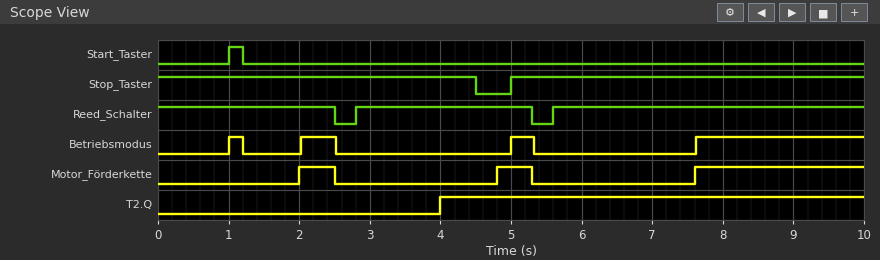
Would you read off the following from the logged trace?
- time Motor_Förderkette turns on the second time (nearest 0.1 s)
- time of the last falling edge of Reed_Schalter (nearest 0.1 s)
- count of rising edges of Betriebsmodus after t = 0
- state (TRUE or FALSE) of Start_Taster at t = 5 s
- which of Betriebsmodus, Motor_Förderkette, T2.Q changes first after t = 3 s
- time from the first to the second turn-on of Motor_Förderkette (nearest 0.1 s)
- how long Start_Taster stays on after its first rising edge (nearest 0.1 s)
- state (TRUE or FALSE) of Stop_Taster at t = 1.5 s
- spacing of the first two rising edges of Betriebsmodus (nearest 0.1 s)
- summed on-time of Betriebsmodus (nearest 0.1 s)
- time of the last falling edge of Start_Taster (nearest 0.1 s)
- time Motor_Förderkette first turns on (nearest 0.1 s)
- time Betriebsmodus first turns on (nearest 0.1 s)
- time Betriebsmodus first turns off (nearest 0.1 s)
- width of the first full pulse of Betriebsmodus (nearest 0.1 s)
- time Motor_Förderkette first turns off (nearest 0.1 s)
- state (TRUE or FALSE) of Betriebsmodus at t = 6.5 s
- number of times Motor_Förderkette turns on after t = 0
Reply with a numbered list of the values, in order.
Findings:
1. 4.8 s
2. 5.3 s
3. 4
4. FALSE
5. T2.Q
6. 2.8 s
7. 0.2 s
8. TRUE
9. 1.0 s
10. 3.4 s
11. 1.2 s
12. 2.0 s
13. 1.0 s
14. 1.2 s
15. 0.2 s
16. 2.5 s
17. FALSE
18. 3
